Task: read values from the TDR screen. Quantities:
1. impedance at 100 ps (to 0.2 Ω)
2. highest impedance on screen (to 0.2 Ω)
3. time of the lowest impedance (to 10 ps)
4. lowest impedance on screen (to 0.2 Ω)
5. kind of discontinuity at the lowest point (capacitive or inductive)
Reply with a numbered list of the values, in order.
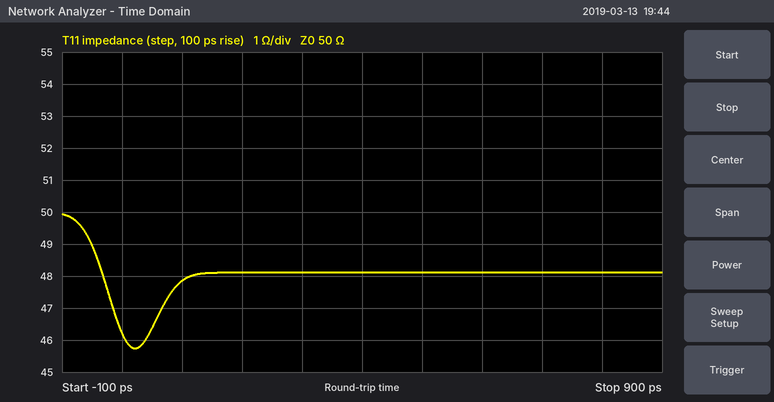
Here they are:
1. 47.8 Ω
2. 50.0 Ω
3. 20 ps
4. 45.8 Ω
5. capacitive
